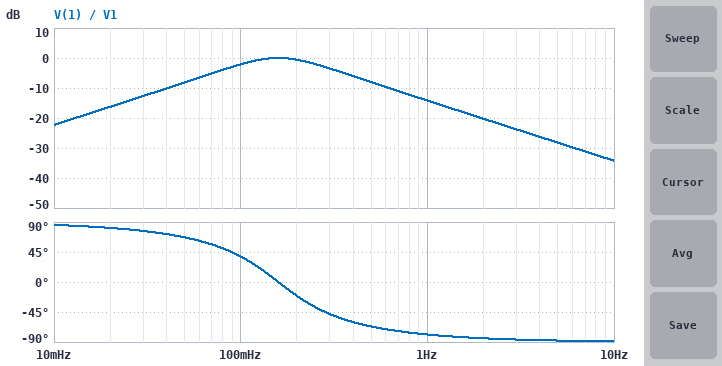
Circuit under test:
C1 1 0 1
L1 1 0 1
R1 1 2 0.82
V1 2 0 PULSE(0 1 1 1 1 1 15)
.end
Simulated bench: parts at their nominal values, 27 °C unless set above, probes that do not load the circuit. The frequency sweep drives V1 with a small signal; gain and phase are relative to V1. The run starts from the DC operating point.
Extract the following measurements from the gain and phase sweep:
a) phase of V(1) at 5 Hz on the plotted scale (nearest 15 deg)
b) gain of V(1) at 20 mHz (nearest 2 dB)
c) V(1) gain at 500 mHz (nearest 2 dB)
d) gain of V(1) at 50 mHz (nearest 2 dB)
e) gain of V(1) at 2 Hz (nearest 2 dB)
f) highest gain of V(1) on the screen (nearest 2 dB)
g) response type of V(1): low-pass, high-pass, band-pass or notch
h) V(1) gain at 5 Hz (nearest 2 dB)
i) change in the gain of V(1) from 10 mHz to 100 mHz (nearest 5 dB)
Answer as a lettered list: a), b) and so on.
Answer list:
a) -90 deg
b) -16 dB
c) -8 dB
d) -8 dB
e) -20 dB
f) 0 dB
g) band-pass
h) -28 dB
i) 20 dB
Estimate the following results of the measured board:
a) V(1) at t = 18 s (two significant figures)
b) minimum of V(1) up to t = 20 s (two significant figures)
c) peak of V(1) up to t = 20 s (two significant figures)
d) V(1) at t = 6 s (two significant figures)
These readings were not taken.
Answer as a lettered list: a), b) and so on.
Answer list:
a) 560 mV
b) -490 mV
c) 580 mV
d) -350 mV
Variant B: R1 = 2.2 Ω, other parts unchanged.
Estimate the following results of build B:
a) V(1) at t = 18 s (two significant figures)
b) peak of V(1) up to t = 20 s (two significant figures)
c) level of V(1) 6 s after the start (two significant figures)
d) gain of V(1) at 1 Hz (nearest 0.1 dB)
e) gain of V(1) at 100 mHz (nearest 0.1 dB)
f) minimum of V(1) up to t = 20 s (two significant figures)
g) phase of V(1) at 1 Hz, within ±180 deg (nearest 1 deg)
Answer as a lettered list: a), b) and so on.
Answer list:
a) 300 mV
b) 320 mV
c) -320 mV
d) -22.6 dB
e) -7.4 dB
f) -390 mV
g) -86 deg
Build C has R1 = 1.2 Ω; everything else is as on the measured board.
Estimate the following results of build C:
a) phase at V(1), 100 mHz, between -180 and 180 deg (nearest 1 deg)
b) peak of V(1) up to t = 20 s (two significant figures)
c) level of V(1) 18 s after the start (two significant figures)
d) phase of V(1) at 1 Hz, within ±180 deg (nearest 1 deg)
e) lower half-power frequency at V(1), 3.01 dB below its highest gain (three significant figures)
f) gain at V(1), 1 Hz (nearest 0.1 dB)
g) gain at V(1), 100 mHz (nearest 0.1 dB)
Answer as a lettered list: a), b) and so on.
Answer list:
a) 49 deg
b) 470 mV
c) 460 mV
d) -82 deg
e) 106 mHz
f) -17.4 dB
g) -3.7 dB
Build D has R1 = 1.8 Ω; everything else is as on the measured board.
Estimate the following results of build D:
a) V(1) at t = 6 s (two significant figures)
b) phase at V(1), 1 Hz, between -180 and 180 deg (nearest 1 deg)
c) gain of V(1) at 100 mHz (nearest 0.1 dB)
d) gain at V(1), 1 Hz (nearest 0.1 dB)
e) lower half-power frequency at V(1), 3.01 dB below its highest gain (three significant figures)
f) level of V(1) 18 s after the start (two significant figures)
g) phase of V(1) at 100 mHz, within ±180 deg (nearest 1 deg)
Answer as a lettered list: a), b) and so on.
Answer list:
a) -340 mV
b) -85 deg
c) -6.0 dB
d) -20.9 dB
e) 121 mHz
f) 350 mV
g) 60 deg
